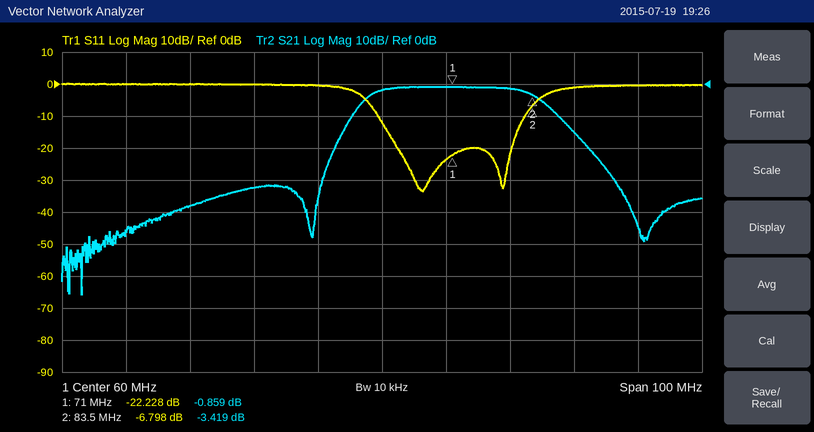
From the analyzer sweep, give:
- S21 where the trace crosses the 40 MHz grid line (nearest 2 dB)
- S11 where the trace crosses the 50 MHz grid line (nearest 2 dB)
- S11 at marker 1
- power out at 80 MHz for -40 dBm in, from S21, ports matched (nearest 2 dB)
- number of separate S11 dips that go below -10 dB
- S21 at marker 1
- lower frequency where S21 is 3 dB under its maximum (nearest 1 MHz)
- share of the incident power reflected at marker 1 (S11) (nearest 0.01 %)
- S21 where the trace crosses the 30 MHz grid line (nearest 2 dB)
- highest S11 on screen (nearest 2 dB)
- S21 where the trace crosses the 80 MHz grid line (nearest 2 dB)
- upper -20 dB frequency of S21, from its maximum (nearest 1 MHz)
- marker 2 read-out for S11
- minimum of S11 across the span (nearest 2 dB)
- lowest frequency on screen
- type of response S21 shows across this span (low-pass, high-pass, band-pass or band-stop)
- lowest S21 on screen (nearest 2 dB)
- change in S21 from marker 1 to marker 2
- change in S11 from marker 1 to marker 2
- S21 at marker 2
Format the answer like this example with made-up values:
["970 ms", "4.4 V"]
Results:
["-32 dB", "0 dB", "-22.228 dB", "-42 dBm", "2", "-0.859 dB", "58 MHz", "0.60 %", "-38 dB", "0 dB", "-2 dB", "93 MHz", "-6.798 dB", "-34 dB", "10 MHz", "band-pass", "-66 dB", "-2.560 dB", "15.430 dB", "-3.419 dB"]
